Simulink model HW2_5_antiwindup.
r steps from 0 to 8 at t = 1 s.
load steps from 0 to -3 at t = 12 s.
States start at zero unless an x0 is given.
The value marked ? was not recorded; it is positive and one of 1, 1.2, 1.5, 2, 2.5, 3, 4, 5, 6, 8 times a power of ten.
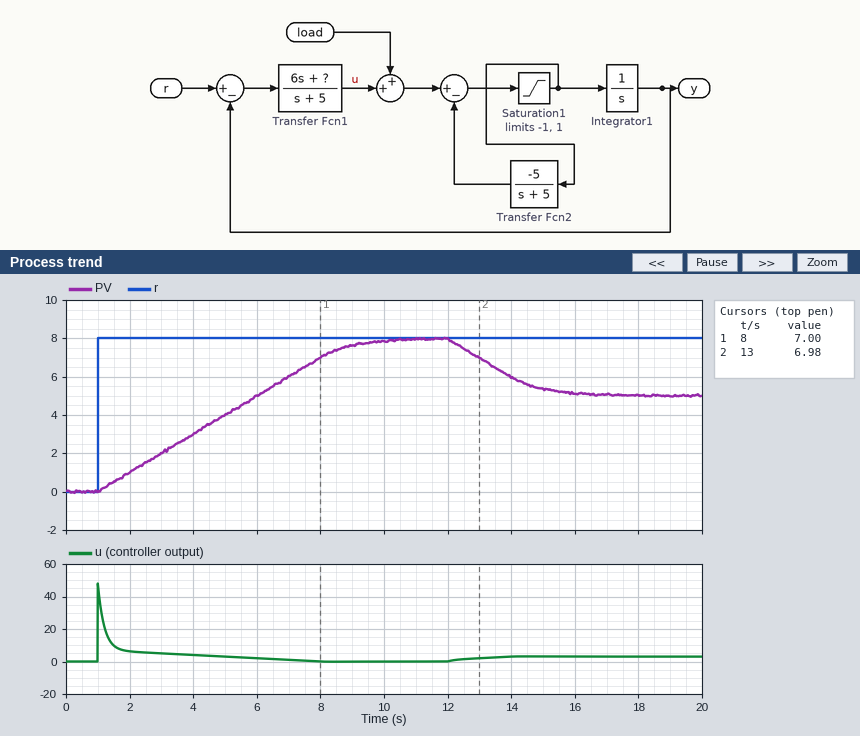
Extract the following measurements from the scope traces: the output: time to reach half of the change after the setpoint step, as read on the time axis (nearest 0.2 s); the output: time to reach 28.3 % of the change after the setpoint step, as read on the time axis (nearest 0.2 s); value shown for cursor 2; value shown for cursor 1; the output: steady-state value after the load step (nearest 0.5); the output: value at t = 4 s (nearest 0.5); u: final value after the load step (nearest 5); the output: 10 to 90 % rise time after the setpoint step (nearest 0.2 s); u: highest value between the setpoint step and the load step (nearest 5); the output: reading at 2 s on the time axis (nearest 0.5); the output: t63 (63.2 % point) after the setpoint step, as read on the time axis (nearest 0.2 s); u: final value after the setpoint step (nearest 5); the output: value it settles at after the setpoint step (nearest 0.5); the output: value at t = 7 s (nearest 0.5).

5.0 s
3.2 s
6.98
7.00
5.0
3.0
5
6.4 s
50
1.0
6.0 s
0
8.0
6.0
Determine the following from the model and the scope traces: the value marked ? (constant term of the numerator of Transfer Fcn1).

5
